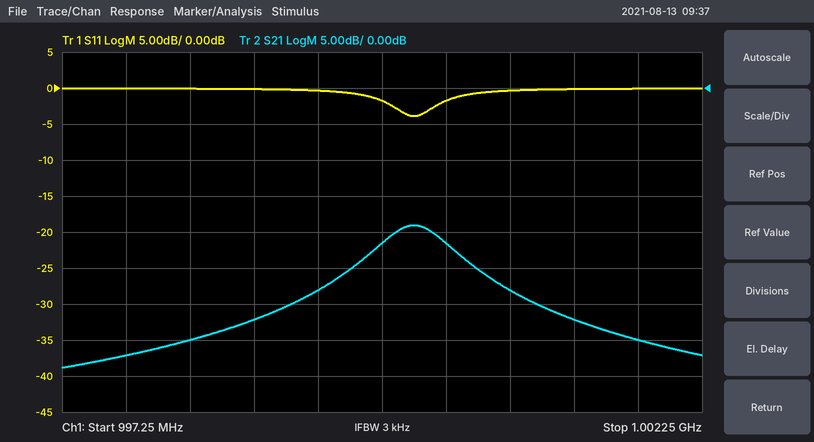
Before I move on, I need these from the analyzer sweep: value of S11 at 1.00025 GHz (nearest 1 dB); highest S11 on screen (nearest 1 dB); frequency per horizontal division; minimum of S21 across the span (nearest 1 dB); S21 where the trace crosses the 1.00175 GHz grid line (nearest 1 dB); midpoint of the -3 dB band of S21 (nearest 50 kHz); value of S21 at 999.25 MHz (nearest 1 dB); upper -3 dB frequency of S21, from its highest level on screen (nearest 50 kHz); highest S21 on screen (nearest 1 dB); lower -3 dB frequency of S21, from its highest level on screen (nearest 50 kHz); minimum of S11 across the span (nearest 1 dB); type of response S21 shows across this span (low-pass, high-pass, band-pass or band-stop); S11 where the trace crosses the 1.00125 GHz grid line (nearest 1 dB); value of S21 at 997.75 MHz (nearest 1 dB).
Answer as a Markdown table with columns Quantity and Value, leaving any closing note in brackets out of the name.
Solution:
| Quantity | Value |
|---|---|
| value of S11 at 1.00025 GHz | -2 dB |
| highest S11 on screen | 0 dB |
| frequency per horizontal division | 500 kHz |
| minimum of S21 across the span | -39 dB |
| S21 where the trace crosses the 1.00175 GHz grid line | -35 dB |
| midpoint of the -3 dB band of S21 | 1.00000 GHz |
| value of S21 at 999.25 MHz | -28 dB |
| upper -3 dB frequency of S21, from its highest level on screen | 1.00030 GHz |
| highest S21 on screen | -19 dB |
| lower -3 dB frequency of S21, from its highest level on screen | 999.70 MHz |
| minimum of S11 across the span | -4 dB |
| type of response S21 shows across this span | band-pass |
| S11 where the trace crosses the 1.00125 GHz grid line | 0 dB |
| value of S21 at 997.75 MHz | -37 dB |
